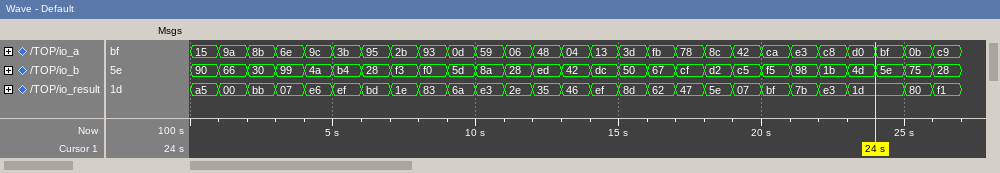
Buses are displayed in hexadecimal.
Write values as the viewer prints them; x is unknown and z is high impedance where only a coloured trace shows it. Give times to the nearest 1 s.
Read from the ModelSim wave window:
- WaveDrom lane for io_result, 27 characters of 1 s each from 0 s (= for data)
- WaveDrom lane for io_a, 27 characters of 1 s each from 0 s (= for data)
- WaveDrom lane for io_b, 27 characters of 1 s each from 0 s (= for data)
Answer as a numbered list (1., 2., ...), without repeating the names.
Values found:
1. {name: 'io_result', wave: '========================.==', data: 'a5 00 bb 07 e6 ef bd 1e 83 6a e3 2e 35 46 ef 8d 62 47 5e 07 bf 7b e3 1d 80 f1'}
2. {name: 'io_a', wave: '===========================', data: '15 9a 8b 6e 9c 3b 95 2b 93 0d 59 06 48 04 13 3d fb 78 8c 42 ca e3 c8 d0 bf 0b c9'}
3. {name: 'io_b', wave: '===========================', data: '90 66 30 99 4a b4 28 f3 f0 5d 8a 28 ed 42 dc 50 67 cf d2 c5 f5 98 1b 4d 5e 75 28'}
